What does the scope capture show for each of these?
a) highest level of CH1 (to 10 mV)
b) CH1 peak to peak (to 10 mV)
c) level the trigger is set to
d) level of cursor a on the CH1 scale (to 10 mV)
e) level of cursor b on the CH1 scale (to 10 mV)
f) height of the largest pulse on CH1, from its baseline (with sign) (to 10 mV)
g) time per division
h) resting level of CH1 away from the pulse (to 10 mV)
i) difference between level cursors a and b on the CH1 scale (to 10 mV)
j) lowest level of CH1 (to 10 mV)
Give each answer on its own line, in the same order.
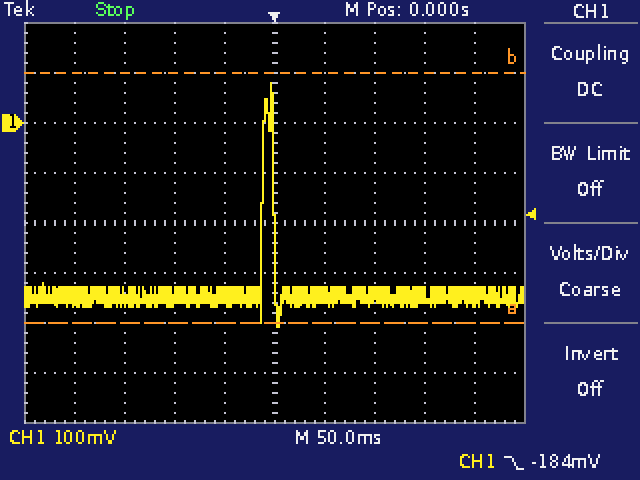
80 mV
490 mV
-184 mV
-400 mV
100 mV
+420 mV
50 ms
-340 mV
500 mV
-410 mV
